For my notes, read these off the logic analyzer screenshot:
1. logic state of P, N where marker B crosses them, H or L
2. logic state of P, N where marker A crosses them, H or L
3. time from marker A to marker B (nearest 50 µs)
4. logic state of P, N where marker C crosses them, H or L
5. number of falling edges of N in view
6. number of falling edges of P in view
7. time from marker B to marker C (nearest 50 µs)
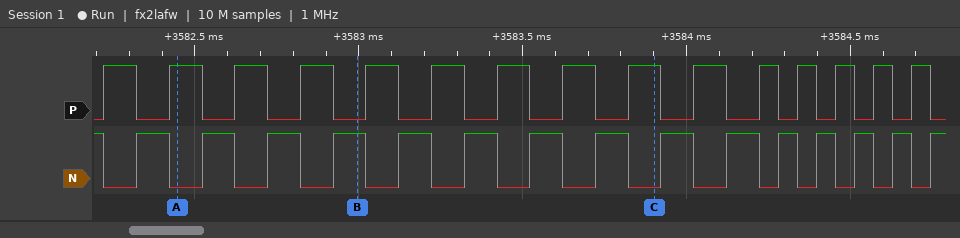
P=L, N=H
P=H, N=L
550 µs
P=H, N=L
15
15
900 µs
